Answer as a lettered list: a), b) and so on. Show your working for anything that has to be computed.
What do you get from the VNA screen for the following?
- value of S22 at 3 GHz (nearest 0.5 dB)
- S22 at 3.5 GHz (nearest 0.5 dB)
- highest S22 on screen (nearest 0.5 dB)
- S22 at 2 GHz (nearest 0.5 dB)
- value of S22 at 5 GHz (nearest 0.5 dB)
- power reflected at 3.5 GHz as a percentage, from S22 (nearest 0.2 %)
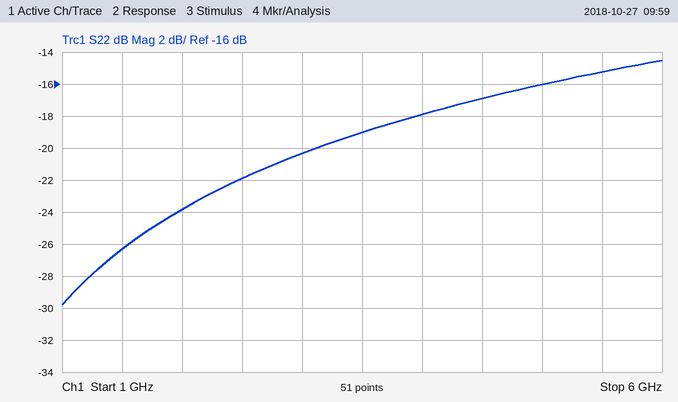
a) -20.5 dB
b) -19.0 dB
c) -14.5 dB
d) -24.0 dB
e) -16.0 dB
f) 10^(-19/10) ≈ 1.26 %, so 1.2 % to the nearest 0.2 %
